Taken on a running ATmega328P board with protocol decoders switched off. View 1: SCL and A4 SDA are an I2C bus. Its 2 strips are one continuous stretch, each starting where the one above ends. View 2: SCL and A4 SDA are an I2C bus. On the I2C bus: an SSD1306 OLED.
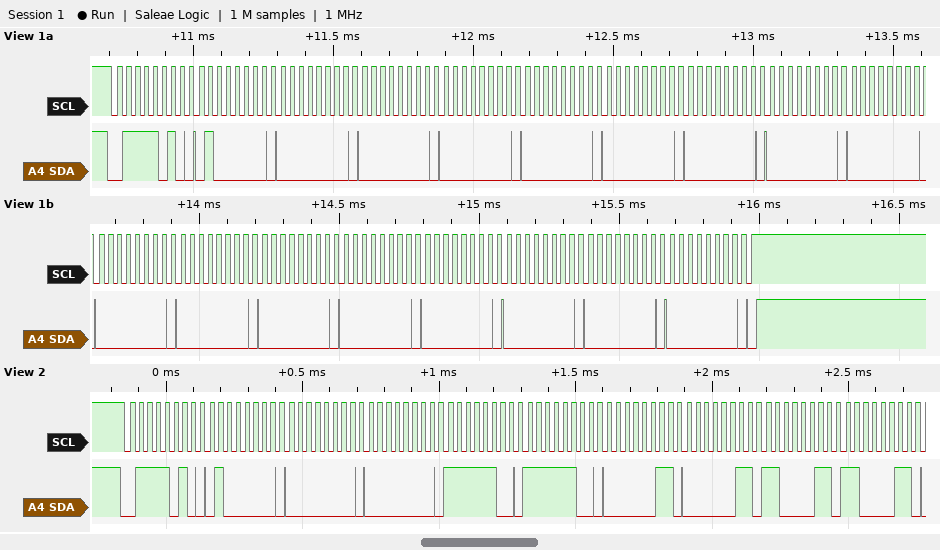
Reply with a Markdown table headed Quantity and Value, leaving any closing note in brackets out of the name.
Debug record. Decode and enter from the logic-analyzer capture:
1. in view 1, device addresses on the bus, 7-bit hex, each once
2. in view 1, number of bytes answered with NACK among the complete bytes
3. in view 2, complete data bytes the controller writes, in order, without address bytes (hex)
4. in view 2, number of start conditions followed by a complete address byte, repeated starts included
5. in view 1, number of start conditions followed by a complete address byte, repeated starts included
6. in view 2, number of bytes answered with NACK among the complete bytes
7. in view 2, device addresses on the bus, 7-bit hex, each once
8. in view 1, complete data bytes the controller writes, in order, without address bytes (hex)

| Quantity | Value |
|---|---|
| in view 1, device addresses on the bus, 7-bit hex, each once | 0x3D |
| in view 1, number of bytes answered with NACK among the complete bytes | 0 |
| in view 2, complete data bytes the controller writes, in order, without address bytes | 40 00 00 FC FC 03 03 C3 C3 |
| in view 2, number of start conditions followed by a complete address byte, repeated starts included | 1 |
| in view 1, number of start conditions followed by a complete address byte, repeated starts included | 1 |
| in view 2, number of bytes answered with NACK among the complete bytes | 0 |
| in view 2, device addresses on the bus, 7-bit hex, each once | 0x3D |
| in view 1, complete data bytes the controller writes, in order, without address bytes | 40 00 00 00 00 00 00 00 00 00 00 00 00 00 00 00 00 |
